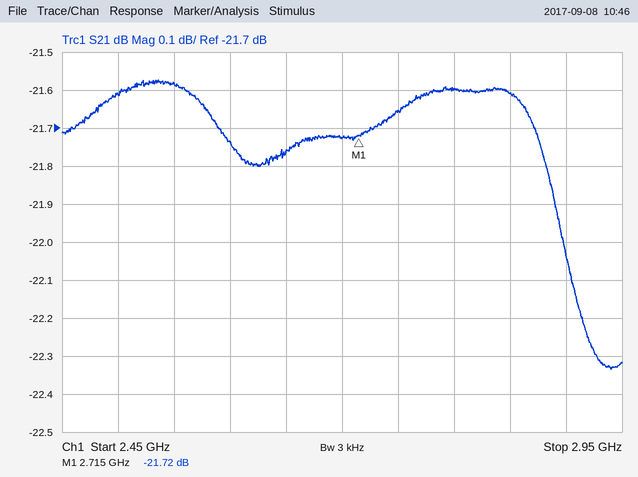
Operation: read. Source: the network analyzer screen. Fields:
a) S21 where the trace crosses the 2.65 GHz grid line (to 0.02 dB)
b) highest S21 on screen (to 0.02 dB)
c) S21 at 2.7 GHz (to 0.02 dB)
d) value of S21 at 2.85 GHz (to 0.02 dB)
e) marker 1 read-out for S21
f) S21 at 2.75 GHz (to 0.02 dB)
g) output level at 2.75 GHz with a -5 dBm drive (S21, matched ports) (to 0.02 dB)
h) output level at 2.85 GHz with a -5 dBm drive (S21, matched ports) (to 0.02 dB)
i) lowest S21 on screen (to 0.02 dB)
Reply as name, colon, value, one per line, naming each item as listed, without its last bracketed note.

S21 where the trace crosses the 2.65 GHz grid line: -21.76 dB
highest S21 on screen: -21.58 dB
S21 at 2.7 GHz: -21.72 dB
value of S21 at 2.85 GHz: -21.60 dB
marker 1 read-out for S21: -21.72 dB
S21 at 2.75 GHz: -21.66 dB
output level at 2.75 GHz with a -5 dBm drive (S21, matched ports): -26.66 dBm
output level at 2.85 GHz with a -5 dBm drive (S21, matched ports): -26.60 dBm
lowest S21 on screen: -22.34 dB
